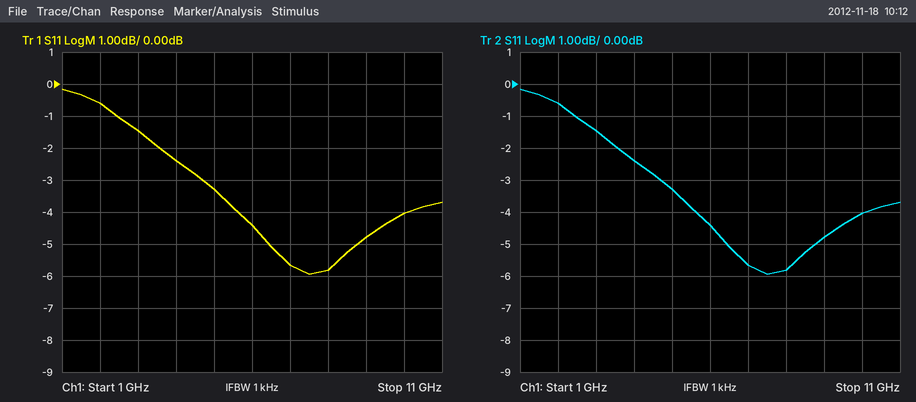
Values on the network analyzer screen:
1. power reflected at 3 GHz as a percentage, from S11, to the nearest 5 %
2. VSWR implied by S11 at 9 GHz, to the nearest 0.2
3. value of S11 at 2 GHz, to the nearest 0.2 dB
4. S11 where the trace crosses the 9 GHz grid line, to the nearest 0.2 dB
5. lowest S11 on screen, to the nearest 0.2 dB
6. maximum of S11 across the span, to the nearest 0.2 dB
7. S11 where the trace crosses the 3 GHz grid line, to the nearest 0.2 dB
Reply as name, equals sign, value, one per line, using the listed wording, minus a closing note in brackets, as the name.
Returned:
power reflected at 3 GHz as a percentage, from S11, to the nearest 5 % = 70 %
VSWR implied by S11 at 9 GHz, to the nearest 0.2 = 3.8
value of S11 at 2 GHz, to the nearest 0.2 dB = -0.6 dB
S11 where the trace crosses the 9 GHz grid line, to the nearest 0.2 dB = -4.8 dB
lowest S11 on screen, to the nearest 0.2 dB = -6.0 dB
maximum of S11 across the span, to the nearest 0.2 dB = -0.2 dB
S11 where the trace crosses the 3 GHz grid line, to the nearest 0.2 dB = -1.4 dB
